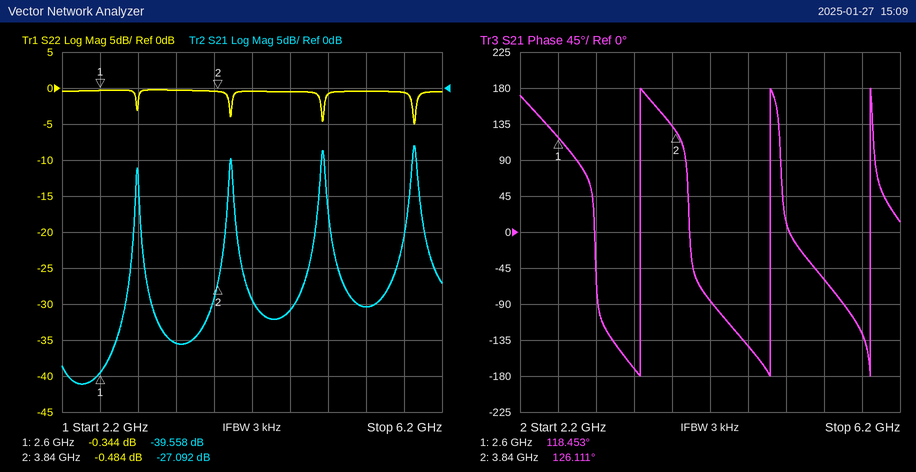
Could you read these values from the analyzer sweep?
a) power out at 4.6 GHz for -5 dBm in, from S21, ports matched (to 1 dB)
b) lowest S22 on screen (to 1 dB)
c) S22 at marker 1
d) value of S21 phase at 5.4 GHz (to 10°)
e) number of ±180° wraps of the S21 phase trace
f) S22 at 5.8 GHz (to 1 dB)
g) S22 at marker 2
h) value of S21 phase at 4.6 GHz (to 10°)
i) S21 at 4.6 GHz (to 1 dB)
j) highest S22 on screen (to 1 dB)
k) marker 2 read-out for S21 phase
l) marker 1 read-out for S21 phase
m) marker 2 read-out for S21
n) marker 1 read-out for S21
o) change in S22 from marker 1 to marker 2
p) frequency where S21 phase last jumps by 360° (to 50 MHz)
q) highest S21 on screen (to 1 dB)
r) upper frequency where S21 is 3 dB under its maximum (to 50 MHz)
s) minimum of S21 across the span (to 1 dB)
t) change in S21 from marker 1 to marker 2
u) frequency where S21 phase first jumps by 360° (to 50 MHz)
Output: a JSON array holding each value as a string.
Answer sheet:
["-36 dBm", "-5 dB", "-0.344 dB", "-60°", "3", "-1 dB", "-0.484 dB", "-140°", "-31 dB", "0 dB", "126.111°", "118.453°", "-27.092 dB", "-39.558 dB", "-0.140 dB", "5.90 GHz", "-8 dB", "5.95 GHz", "-41 dB", "12.466 dB", "3.45 GHz"]
